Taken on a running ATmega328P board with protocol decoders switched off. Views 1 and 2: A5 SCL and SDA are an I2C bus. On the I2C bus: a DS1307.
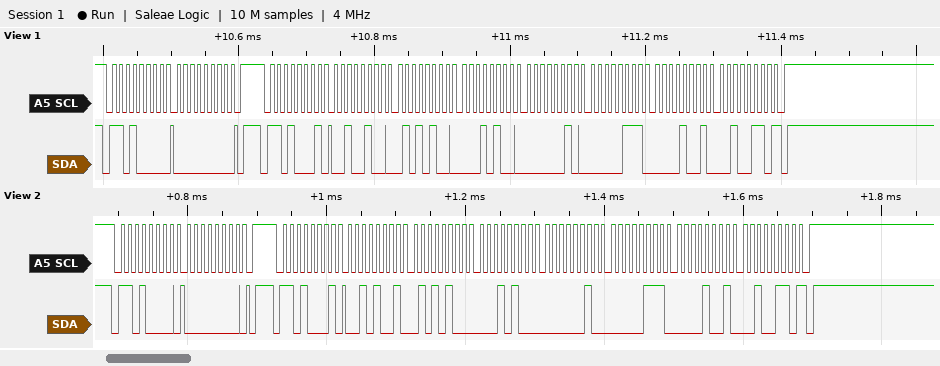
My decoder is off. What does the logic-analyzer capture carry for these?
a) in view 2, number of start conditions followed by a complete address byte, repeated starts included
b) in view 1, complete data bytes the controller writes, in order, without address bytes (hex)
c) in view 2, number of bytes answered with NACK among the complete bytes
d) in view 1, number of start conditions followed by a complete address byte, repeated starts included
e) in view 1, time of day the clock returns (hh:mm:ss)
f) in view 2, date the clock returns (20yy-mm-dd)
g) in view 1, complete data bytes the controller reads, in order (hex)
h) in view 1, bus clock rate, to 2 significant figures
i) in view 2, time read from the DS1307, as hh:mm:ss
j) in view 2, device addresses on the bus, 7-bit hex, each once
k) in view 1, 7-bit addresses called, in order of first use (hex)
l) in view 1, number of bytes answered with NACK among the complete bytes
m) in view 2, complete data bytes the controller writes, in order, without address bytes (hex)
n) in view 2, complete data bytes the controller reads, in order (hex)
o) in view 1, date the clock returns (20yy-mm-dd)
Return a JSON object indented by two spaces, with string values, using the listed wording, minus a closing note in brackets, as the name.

{
  "in view 2, number of start conditions followed by a complete address byte, repeated starts included": "2",
  "in view 1, complete data bytes the controller writes, in order, without address bytes": "00",
  "in view 2, number of bytes answered with NACK among the complete bytes": "1",
  "in view 1, number of start conditions followed by a complete address byte, repeated starts included": "2",
  "in view 1, time of day the clock returns": "14:54:24",
  "in view 2, date the clock returns": "2026-09-07",
  "in view 1, complete data bytes the controller reads, in order": "24 54 14 02 07 09 26",
  "in view 1, bus clock rate, to 2 significant figures": "100 kHz",
  "in view 2, time read from the DS1307, as hh:mm:ss": "14:54:29",
  "in view 2, device addresses on the bus, 7-bit hex, each once": "0x68",
  "in view 1, 7-bit addresses called, in order of first use": "0x68",
  "in view 1, number of bytes answered with NACK among the complete bytes": "1",
  "in view 2, complete data bytes the controller writes, in order, without address bytes": "00",
  "in view 2, complete data bytes the controller reads, in order": "29 54 14 02 07 09 26",
  "in view 1, date the clock returns": "2026-09-07"
}
